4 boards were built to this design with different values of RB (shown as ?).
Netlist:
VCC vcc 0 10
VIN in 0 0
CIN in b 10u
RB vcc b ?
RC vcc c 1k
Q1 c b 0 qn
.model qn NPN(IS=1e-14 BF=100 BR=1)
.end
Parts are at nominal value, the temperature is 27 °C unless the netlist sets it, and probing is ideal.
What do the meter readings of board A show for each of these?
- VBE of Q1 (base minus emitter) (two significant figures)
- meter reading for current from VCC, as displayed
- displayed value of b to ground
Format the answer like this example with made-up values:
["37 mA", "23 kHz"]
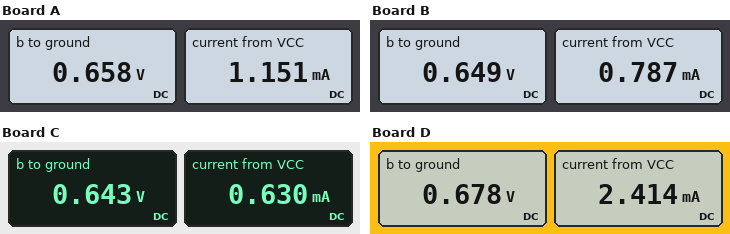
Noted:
["660 mV", "1.151 mA", "0.658 V"]
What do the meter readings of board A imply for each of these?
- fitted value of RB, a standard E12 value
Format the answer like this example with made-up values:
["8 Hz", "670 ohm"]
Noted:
["820 kΩ"]
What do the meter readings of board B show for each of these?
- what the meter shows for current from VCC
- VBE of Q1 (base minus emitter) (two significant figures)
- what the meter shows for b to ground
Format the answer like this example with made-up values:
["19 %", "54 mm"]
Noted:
["0.787 mA", "650 mV", "0.649 V"]
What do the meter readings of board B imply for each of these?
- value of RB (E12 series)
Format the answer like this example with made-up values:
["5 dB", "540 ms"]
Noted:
["1.2 MΩ"]
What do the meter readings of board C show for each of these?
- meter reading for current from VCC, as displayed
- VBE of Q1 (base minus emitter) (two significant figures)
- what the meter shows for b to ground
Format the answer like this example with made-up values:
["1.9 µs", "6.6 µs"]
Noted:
["0.630 mA", "640 mV", "0.643 V"]
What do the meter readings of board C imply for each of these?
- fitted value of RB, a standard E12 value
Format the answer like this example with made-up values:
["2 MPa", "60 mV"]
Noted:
["1.5 MΩ"]
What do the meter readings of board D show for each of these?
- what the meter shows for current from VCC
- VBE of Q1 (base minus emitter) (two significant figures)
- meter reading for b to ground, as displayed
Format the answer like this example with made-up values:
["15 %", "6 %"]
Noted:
["2.414 mA", "680 mV", "0.678 V"]
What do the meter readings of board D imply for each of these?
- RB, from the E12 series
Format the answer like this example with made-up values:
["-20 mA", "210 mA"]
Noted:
["390 kΩ"]
